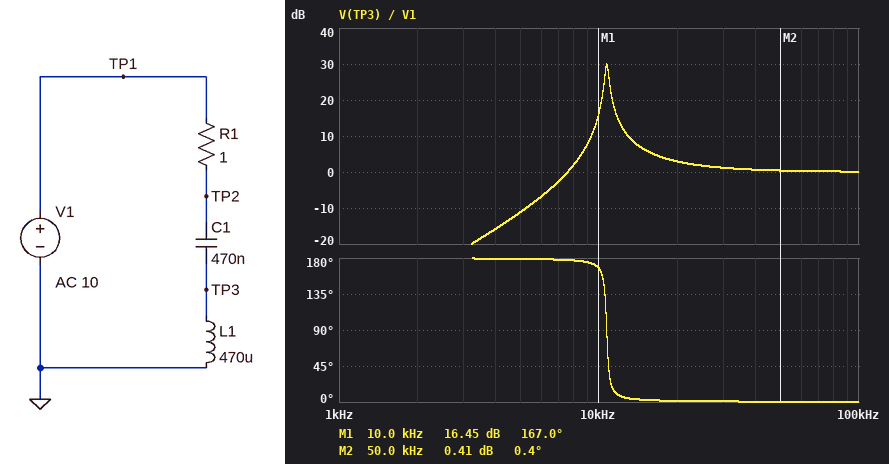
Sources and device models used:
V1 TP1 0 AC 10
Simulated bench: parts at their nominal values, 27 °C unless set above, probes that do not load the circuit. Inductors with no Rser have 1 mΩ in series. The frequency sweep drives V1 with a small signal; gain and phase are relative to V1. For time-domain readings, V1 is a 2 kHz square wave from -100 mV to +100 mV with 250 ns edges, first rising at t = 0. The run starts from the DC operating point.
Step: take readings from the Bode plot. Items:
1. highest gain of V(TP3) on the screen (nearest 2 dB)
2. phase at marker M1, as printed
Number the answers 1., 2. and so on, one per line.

1. 30 dB
2. 167.0 deg
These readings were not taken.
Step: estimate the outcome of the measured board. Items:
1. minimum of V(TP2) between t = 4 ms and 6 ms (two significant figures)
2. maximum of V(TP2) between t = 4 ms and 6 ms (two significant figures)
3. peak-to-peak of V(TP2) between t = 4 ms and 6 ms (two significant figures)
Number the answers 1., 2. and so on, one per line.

1. -110 mV
2. 110 mV
3. 210 mV
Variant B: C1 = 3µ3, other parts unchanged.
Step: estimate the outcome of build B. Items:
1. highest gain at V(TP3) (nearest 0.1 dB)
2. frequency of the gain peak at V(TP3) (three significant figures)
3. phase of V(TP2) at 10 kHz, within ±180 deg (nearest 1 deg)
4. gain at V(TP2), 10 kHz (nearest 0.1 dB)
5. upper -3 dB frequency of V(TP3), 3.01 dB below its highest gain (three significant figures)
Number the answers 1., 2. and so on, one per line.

1. 21.5 dB
2. 4.05 kHz
3. 2 deg
4. 0 dB
5. 4.23 kHz
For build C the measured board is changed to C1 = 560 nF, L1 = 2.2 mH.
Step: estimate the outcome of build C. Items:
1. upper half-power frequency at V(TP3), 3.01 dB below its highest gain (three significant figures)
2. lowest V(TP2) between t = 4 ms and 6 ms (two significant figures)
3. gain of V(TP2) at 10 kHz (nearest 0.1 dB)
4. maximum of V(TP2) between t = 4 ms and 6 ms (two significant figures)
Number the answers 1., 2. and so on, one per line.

1. 4.57 kHz
2. -100 mV
3. 0 dB
4. 100 mV
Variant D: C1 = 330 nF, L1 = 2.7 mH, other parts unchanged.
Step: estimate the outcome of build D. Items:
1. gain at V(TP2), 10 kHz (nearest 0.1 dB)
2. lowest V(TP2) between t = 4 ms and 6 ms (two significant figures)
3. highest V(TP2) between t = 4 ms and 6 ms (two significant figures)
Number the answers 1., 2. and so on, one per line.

1. 0 dB
2. -100 mV
3. 100 mV
